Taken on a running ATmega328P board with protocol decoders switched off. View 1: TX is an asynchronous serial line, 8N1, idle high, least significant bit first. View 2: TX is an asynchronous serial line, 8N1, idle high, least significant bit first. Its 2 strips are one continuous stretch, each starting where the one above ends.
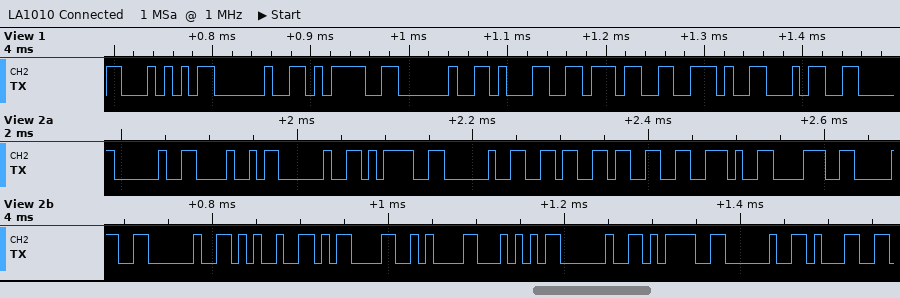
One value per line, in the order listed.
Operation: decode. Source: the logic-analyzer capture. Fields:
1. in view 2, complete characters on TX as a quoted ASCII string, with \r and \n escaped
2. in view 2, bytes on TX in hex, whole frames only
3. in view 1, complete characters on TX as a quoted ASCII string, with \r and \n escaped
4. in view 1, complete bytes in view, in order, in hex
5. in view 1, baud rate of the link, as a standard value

" H = 63.80 %\r\nT = 1"
20 48 20 3D 20 36 33 2E 38 30 20 25 0D 0A 54 20 3D 20 31
"T = 17.4"
54 20 3D 20 31 37 2E 34
115200 baud
